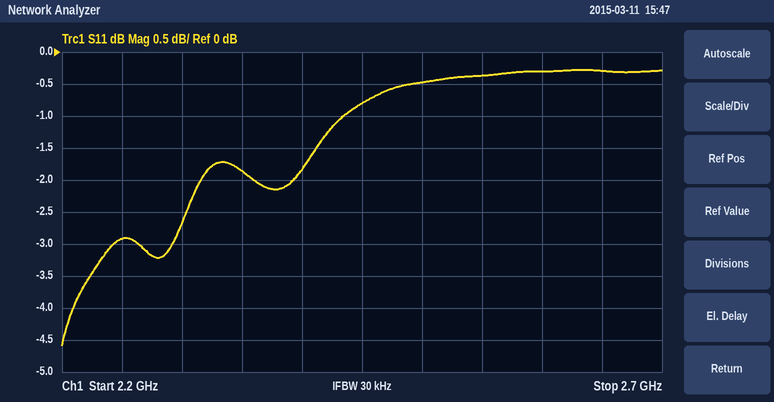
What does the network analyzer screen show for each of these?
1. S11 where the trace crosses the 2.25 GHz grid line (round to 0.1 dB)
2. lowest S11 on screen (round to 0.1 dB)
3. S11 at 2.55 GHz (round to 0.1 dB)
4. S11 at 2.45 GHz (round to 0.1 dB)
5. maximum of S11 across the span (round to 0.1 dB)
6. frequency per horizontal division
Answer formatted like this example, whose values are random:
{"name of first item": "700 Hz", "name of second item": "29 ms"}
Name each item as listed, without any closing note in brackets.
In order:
{"S11 where the trace crosses the 2.25 GHz grid line": "-2.9 dB", "lowest S11 on screen": "-4.6 dB", "S11 at 2.55 GHz": "-0.4 dB", "S11 at 2.45 GHz": "-0.8 dB", "maximum of S11 across the span": "-0.3 dB", "frequency per horizontal division": "50 MHz"}
